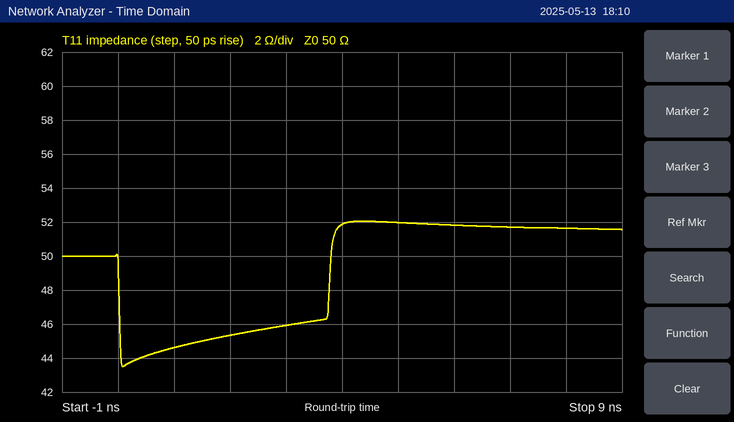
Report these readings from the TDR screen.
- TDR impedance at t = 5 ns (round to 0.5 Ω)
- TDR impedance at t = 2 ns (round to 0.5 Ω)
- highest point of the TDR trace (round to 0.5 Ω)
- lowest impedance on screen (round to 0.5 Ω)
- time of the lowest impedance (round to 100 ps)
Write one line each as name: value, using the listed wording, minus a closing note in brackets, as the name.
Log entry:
TDR impedance at t = 5 ns: 52.0 Ω
TDR impedance at t = 2 ns: 45.5 Ω
highest point of the TDR trace: 52.0 Ω
lowest impedance on screen: 43.5 Ω
time of the lowest impedance: 100 ps
